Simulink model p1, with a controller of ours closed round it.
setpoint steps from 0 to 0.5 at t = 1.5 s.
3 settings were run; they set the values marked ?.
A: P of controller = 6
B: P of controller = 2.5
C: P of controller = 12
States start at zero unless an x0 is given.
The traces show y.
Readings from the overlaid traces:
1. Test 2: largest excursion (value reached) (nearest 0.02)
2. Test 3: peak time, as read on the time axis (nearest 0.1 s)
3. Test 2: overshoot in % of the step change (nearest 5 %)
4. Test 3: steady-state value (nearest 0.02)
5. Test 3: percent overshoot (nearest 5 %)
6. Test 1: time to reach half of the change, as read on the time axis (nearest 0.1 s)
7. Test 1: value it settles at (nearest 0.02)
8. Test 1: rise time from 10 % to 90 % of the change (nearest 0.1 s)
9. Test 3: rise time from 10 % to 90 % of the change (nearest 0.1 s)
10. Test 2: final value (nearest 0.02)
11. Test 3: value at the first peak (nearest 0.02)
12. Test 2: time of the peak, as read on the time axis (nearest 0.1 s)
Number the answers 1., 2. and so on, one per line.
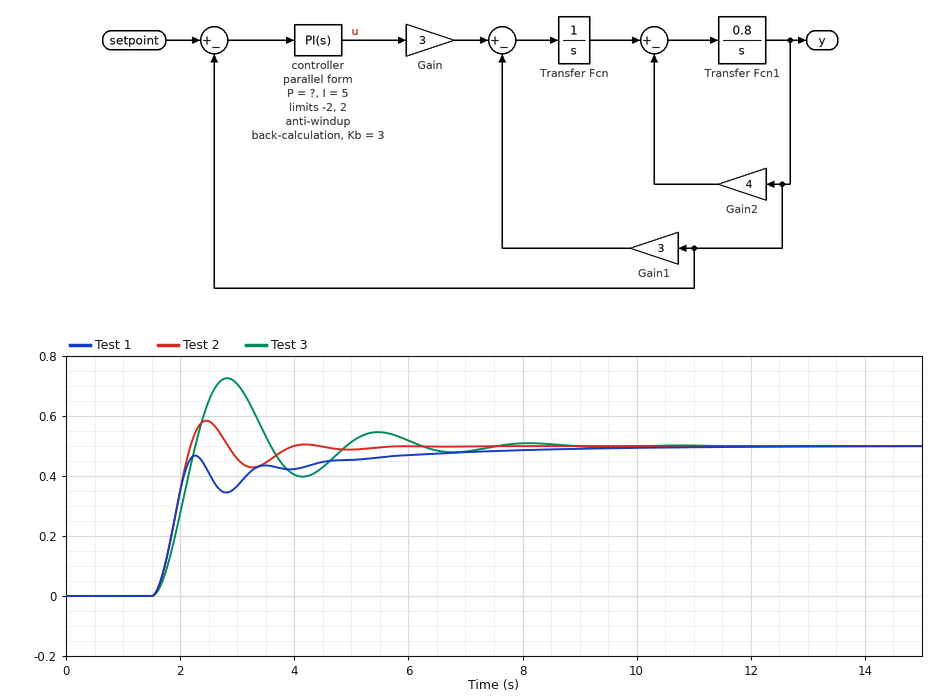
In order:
1. 0.58
2. 2.8 s
3. 15 %
4. 0.50
5. 45 %
6. 1.9 s
7. 0.50
8. 0.5 s
9. 0.5 s
10. 0.50
11. 0.72
12. 2.5 s
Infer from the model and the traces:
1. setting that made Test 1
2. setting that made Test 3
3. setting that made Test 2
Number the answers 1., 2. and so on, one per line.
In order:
1. C
2. B
3. A
